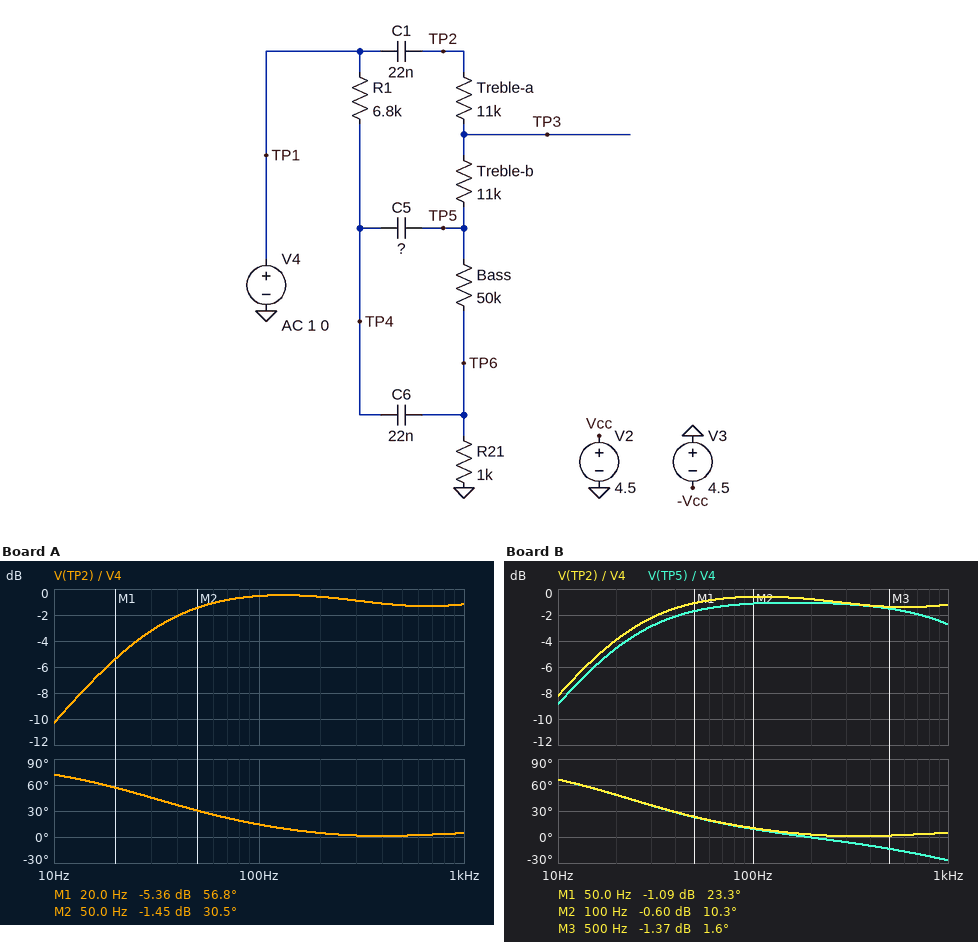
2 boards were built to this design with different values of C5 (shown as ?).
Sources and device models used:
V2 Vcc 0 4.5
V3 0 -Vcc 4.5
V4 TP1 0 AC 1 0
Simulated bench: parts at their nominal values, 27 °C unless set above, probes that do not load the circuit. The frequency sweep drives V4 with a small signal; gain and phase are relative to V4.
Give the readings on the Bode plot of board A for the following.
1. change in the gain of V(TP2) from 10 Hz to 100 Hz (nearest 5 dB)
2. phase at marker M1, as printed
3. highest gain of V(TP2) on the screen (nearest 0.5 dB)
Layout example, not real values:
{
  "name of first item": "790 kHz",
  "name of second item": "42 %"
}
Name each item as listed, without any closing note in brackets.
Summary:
{
  "change in the gain of V(TP2) from 10 Hz to 100 Hz": "10 dB",
  "phase at marker M1, as printed": "56.8 deg",
  "highest gain of V(TP2) on the screen": "-0.5 dB"
}
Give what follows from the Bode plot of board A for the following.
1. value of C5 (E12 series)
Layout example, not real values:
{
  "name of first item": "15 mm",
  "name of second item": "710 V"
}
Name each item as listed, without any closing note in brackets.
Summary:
{
  "value of C5": "68 nF"
}
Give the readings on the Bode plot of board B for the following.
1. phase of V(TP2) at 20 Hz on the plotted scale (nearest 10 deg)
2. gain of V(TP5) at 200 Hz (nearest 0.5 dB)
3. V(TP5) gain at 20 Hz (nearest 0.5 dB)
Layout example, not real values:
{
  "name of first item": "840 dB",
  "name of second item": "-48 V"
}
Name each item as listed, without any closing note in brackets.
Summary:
{
  "phase of V(TP2) at 20 Hz on the plotted scale": "50 deg",
  "gain of V(TP5) at 200 Hz": "-1.0 dB",
  "V(TP5) gain at 20 Hz": "-4.5 dB"
}
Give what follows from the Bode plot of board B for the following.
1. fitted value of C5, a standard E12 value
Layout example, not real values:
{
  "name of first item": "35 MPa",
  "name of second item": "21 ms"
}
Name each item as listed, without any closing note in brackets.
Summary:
{
  "fitted value of C5, a standard E12 value": "100 nF"
}
